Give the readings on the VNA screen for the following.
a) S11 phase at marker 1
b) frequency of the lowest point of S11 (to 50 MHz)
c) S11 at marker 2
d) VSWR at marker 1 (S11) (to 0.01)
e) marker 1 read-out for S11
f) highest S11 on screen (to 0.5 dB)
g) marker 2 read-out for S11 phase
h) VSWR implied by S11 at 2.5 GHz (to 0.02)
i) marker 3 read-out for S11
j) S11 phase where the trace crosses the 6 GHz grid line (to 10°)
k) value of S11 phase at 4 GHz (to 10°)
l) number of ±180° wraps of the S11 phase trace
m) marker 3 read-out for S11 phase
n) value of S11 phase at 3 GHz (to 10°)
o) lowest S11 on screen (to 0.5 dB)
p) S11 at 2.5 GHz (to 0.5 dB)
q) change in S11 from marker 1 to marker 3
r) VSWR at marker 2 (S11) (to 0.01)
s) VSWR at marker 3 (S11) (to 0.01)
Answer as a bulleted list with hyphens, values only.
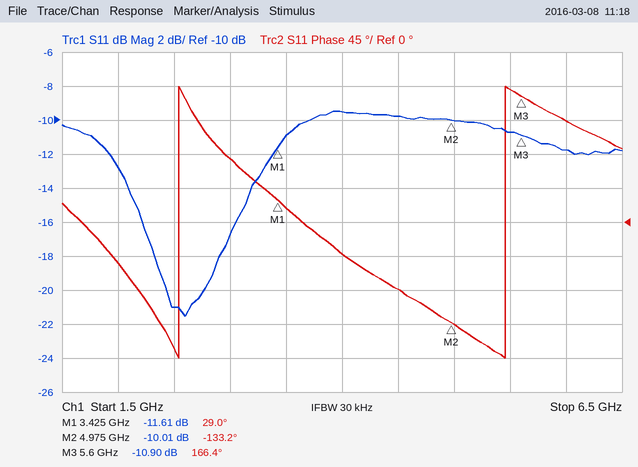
- 29.0°
- 2.60 GHz
- -10.01 dB
- 1.71
- -11.61 dB
- -9.5 dB
- -133.2°
- 1.20
- -10.90 dB
- 130°
- -40°
- 2
- 166.4°
- 80°
- -21.5 dB
- -21.0 dB
- 0.71 dB
- 1.92
- 1.80
